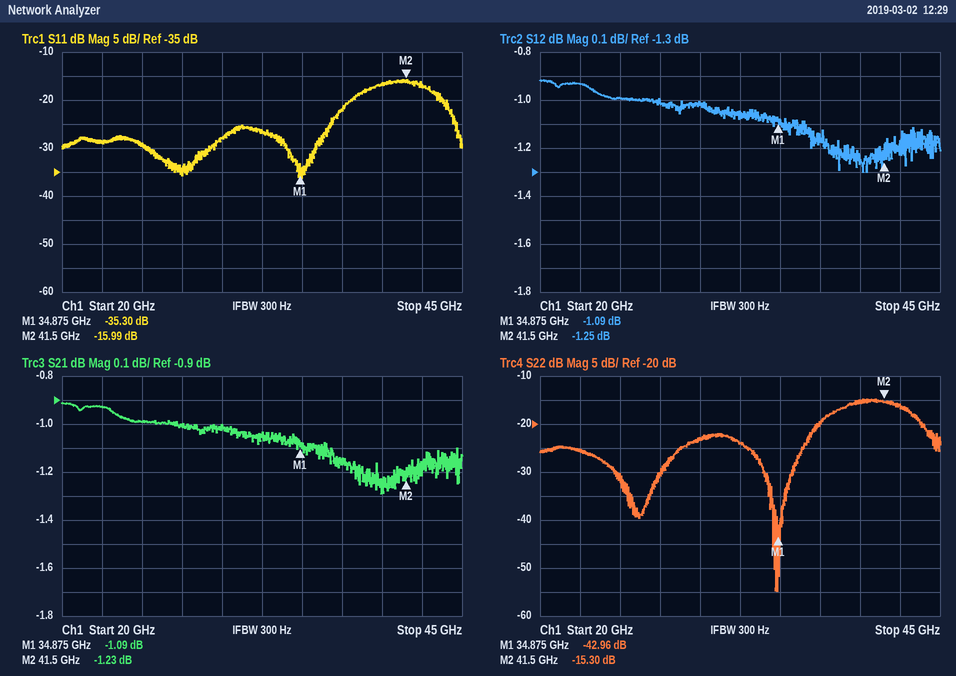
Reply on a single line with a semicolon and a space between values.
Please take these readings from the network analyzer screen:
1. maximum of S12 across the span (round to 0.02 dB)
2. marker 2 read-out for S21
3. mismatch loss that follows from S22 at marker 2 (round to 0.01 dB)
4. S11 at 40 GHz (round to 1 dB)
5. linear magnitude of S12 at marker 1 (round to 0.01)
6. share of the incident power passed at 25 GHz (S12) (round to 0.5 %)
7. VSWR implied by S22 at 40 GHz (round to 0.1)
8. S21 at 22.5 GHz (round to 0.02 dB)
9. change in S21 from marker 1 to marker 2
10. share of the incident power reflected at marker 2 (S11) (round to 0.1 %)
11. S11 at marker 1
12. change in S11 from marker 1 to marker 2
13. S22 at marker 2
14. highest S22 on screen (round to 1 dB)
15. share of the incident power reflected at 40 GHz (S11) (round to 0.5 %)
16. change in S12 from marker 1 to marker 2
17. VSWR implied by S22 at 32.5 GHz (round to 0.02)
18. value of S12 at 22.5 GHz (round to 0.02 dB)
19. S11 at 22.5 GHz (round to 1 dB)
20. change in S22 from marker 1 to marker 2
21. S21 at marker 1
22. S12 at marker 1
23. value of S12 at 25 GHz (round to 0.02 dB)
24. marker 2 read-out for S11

-0.92 dB; -1.23 dB; 0.13 dB; -17 dB; 0.88; 79.5 %; 1.4; -0.92 dB; -0.14 dB; 2.5 %; -35.30 dB; 19.31 dB; -15.30 dB; -15 dB; 2.0 %; -0.16 dB; 1.14; -0.94 dB; -29 dB; 27.66 dB; -1.09 dB; -1.09 dB; -1.00 dB; -15.99 dB
